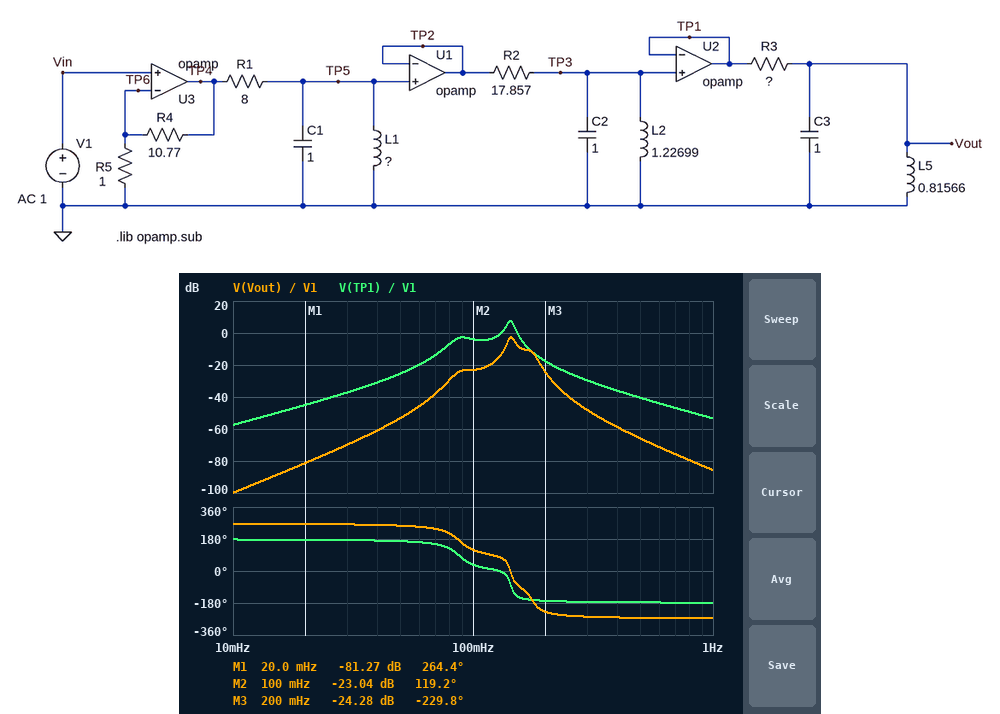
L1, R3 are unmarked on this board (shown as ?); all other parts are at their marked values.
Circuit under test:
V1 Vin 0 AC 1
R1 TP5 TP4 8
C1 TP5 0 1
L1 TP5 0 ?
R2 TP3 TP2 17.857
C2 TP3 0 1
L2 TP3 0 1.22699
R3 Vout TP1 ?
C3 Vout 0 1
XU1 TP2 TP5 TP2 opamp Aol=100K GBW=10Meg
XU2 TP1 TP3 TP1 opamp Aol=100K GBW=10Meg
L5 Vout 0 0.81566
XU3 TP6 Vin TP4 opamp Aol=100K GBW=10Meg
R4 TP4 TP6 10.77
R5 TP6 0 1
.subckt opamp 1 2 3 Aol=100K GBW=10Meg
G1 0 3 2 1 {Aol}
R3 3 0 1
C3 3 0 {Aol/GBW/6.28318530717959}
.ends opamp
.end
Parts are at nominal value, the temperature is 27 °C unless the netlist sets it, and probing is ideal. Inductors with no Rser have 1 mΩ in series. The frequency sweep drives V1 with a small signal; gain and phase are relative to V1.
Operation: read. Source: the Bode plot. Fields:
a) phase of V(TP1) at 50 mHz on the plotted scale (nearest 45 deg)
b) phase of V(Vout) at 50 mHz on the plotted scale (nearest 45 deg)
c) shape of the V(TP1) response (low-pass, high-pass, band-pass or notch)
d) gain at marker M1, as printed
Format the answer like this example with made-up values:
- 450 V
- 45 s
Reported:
- 180 deg
- 270 deg
- band-pass
- -81.27 dB
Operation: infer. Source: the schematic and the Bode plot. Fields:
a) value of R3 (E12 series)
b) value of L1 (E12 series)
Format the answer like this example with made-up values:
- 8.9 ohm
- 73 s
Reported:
- 6.8 Ω
- 3.3 H
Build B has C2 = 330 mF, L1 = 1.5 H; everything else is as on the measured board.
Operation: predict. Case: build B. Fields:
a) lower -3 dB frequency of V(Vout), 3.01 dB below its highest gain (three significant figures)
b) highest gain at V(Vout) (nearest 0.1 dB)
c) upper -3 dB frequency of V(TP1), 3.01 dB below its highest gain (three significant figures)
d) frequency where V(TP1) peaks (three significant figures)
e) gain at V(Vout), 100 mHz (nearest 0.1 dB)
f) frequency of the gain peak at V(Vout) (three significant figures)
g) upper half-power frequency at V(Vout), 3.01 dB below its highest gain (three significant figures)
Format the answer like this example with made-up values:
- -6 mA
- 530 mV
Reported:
- 163 mHz
- -7.6 dB
- 262 mHz
- 249 mHz
- -34.7 dB
- 176 mHz
- 189 mHz
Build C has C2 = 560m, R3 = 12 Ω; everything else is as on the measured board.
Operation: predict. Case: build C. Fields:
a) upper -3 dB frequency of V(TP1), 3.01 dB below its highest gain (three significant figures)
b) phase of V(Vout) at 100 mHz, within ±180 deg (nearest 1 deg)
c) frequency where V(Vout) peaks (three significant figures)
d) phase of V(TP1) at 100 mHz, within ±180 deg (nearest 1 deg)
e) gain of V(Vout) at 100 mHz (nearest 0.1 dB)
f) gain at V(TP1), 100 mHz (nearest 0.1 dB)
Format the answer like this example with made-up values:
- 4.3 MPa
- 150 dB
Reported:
- 199 mHz
- 123 deg
- 179 mHz
- 37 deg
- -30.9 dB
- -6.9 dB
